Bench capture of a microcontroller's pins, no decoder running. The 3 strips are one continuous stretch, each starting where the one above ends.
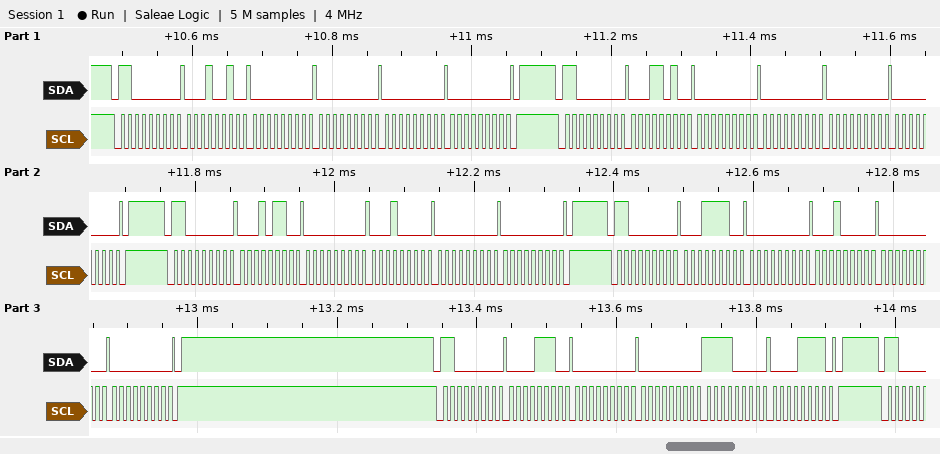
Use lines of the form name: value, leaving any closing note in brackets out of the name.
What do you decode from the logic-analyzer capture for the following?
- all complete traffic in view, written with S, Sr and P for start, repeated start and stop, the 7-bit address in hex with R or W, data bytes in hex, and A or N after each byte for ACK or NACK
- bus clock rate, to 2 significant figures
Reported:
all complete traffic in view, written with S, Sr and P for start, repeated start and stop, the 7-bit address in hex with R or W, data bytes in hex, and A or N after each byte for ACK or NACK: S 60W A 12 A 00 A 00 A 00 A 00 A P S 60W A 1A A 00 A 00 A 00 A 00 A P S 60W A 16 A 00 A 10 A 00 A 00 A P S 60W A 1E A 00 A 10 A 00 A 00 A P S 60W A 0E A 00 A 00 A F0 A 0F A P
bus clock rate, to 2 significant figures: 100 kHz
